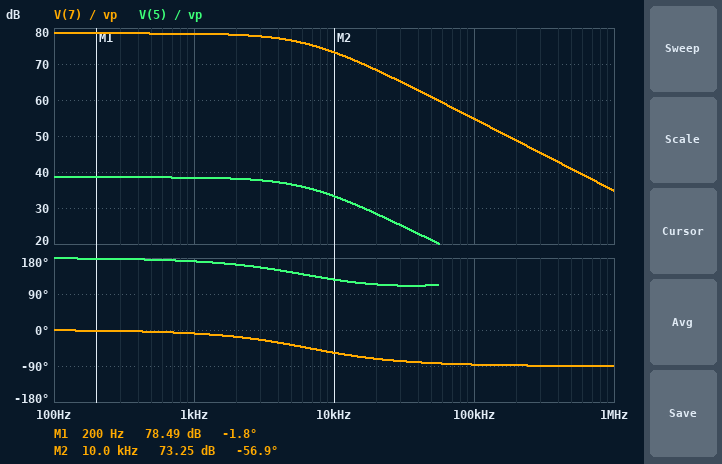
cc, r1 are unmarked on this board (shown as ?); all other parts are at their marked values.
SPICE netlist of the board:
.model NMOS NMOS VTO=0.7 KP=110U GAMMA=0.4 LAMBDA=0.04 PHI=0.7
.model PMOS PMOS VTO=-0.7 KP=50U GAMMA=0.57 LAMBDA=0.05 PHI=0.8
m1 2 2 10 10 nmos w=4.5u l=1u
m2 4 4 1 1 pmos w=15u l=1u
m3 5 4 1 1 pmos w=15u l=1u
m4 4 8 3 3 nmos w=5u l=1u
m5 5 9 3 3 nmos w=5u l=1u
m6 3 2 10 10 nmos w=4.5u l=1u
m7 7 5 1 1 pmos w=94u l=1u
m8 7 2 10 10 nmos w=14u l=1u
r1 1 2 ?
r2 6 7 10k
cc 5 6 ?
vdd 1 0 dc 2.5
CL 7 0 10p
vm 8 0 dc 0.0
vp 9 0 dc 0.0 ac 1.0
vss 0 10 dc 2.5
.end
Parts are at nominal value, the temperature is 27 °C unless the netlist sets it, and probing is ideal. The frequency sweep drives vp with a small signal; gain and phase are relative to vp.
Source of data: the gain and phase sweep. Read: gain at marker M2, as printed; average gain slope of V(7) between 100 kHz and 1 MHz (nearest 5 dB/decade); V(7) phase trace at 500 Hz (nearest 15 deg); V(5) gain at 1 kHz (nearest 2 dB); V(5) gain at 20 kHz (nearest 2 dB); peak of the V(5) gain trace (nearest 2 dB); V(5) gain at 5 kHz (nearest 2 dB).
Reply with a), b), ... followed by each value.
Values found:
a) 73.25 dB
b) -20 dB/decade
c) 0 deg
d) 38 dB
e) 28 dB
f) 38 dB
g) 36 dB
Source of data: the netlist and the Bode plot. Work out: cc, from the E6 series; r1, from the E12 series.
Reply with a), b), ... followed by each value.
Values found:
a) 470 fF
b) 82 kΩ
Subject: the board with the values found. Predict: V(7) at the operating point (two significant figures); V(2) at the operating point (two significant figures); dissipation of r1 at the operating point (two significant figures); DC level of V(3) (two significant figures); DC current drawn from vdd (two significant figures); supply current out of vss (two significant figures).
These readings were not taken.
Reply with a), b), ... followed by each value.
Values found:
a) 520 mV
b) -1.4 V
c) 180 µW
d) -980 mV
e) 250 µA
f) 250 µA
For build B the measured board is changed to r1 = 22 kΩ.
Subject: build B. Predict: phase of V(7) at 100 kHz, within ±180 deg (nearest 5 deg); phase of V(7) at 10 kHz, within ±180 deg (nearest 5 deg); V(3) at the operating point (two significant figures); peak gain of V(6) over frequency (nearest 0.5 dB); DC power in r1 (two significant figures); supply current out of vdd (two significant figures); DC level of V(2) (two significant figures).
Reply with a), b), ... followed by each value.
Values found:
a) -70 deg
b) -15 deg
c) -1.2 V
d) 68.0 dB
e) 560 µW
f) 840 µA
g) -1.0 V
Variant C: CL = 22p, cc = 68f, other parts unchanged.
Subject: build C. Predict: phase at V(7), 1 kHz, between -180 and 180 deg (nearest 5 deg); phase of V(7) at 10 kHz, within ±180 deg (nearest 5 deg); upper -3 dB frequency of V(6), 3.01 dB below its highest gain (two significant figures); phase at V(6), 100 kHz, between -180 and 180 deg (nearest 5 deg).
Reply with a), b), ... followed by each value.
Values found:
a) 0 deg
b) -20 deg
c) 31 kHz
d) -75 deg
